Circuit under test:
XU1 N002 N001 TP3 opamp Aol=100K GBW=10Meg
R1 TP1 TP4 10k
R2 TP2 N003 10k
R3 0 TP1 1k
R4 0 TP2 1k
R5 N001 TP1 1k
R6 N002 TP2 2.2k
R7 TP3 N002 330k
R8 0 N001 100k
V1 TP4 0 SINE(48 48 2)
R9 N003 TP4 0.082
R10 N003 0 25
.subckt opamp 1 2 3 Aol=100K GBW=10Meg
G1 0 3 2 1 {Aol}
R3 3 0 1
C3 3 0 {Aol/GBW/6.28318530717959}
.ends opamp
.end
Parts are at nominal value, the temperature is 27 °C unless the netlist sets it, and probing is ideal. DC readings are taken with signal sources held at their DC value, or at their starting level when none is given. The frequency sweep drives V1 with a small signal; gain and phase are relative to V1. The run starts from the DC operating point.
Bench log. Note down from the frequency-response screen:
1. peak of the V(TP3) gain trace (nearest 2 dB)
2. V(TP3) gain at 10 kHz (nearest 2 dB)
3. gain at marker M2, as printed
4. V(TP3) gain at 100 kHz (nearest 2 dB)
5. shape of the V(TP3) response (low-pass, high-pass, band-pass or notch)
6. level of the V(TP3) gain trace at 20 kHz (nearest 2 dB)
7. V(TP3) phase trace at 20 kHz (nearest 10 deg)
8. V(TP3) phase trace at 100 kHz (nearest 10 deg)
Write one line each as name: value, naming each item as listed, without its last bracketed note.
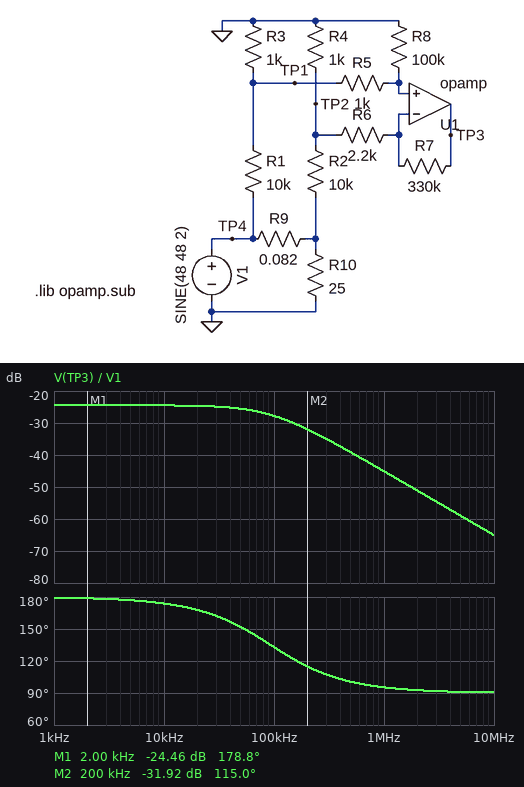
peak of the V(TP3) gain trace: -24 dB
V(TP3) gain at 10 kHz: -24 dB
gain at marker M2, as printed: -31.92 dB
V(TP3) gain at 100 kHz: -28 dB
shape of the V(TP3) response: low-pass
level of the V(TP3) gain trace at 20 kHz: -24 dB
V(TP3) phase trace at 20 kHz: 170 deg
V(TP3) phase trace at 100 kHz: 130 deg
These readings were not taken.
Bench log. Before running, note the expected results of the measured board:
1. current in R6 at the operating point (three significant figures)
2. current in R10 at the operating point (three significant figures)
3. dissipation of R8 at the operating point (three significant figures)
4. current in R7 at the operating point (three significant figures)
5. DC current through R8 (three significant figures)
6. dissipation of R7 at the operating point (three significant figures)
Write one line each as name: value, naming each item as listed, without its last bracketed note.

current in R6 at the operating point: 21.7 µA
current in R10 at the operating point: 1.91 A
dissipation of R8 at the operating point: 183 µW
current in R7 at the operating point: 21.7 µA
DC current through R8: 42.8 µA
dissipation of R7 at the operating point: 155 µW
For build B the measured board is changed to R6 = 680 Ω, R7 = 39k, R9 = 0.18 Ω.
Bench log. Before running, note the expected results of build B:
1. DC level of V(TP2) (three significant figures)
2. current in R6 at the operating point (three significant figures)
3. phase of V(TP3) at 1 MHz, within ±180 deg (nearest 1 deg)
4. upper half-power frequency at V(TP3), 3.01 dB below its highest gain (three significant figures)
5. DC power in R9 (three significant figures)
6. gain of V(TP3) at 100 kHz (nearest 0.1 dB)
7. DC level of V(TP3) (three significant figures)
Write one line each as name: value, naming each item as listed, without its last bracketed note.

DC level of V(TP2): 4.30 V
current in R6 at the operating point: 31.8 µA
phase of V(TP3) at 1 MHz, within ±180 deg: -69 deg
upper half-power frequency at V(TP3), 3.01 dB below its highest gain: 392 kHz
DC power in R9: 657 mW
gain of V(TP3) at 100 kHz: -24.2 dB
DC level of V(TP3): 3.04 V
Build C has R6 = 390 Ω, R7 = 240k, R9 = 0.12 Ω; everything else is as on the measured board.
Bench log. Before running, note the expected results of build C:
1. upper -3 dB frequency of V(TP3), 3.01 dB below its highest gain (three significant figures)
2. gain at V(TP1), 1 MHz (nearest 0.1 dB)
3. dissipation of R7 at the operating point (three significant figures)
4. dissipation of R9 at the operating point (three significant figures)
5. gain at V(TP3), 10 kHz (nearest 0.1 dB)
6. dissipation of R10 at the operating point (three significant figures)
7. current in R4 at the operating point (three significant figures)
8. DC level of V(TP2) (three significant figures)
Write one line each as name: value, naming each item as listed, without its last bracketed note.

upper -3 dB frequency of V(TP3), 3.01 dB below its highest gain: 53.9 kHz
gain at V(TP1), 1 MHz: -20.9 dB
dissipation of R7 at the operating point: 525 µW
dissipation of R9 at the operating point: 440 mW
gain at V(TP3), 10 kHz: -16.9 dB
dissipation of R10 at the operating point: 91.3 W
current in R4 at the operating point: 4.30 mA
DC level of V(TP2): 4.30 V
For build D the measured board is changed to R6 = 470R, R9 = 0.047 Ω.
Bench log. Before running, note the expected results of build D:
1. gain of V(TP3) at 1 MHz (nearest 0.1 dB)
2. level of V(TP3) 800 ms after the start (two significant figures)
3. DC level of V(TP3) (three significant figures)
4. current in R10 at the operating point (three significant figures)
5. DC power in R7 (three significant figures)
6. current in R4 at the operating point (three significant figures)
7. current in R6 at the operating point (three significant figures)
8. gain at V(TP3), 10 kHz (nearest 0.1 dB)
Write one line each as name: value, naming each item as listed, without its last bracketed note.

gain of V(TP3) at 1 MHz: -38.8 dB
level of V(TP3) 800 ms after the start: -5.5 V
DC level of V(TP3): -13.3 V
current in R10 at the operating point: 1.92 A
DC power in R7: 935 µW
current in R4 at the operating point: 4.31 mA
current in R6 at the operating point: 53.2 µA
gain at V(TP3), 10 kHz: -11.4 dB
